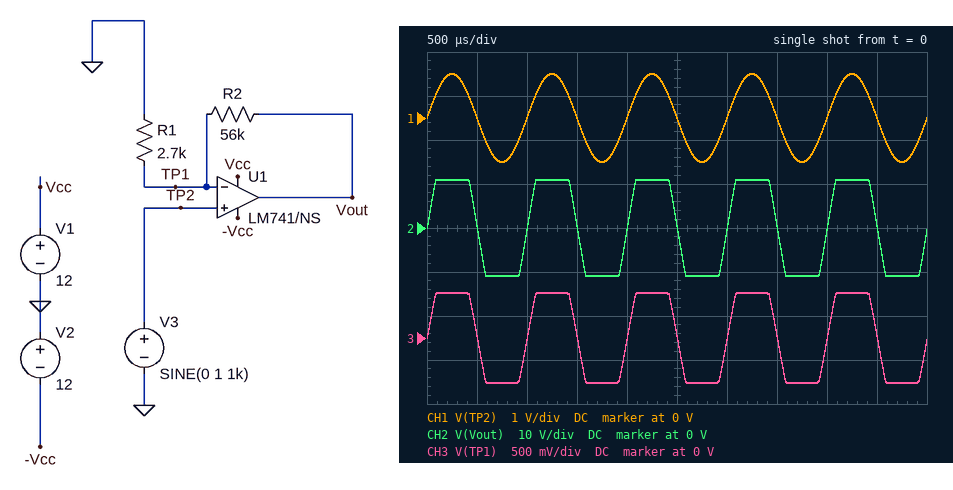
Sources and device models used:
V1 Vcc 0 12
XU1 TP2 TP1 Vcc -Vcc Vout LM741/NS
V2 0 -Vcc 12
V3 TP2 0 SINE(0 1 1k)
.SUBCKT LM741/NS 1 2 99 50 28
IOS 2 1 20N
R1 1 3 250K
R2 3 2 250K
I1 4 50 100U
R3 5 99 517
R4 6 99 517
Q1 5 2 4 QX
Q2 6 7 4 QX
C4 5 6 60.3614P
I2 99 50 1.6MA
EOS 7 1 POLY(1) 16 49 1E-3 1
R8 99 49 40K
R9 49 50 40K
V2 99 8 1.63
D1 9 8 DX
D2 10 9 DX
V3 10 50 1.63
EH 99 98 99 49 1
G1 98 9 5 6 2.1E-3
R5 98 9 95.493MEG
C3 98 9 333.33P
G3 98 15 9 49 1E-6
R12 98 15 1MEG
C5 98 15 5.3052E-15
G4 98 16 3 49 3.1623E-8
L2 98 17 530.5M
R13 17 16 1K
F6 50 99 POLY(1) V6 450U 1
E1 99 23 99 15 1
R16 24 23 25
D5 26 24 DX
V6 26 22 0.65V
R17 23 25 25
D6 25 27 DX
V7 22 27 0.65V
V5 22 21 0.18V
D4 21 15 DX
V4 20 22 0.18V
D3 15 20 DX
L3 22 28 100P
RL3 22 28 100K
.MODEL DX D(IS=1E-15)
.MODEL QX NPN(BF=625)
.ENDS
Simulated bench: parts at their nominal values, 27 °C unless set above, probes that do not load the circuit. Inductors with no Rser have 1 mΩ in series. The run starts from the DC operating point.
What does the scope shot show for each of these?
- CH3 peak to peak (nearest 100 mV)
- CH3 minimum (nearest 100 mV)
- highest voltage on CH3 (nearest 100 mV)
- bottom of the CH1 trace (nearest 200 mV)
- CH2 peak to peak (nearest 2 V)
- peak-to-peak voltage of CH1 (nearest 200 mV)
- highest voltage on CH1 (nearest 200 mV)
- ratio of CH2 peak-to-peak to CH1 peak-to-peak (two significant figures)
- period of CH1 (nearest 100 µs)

1.0 V
-500 mV
500 mV
-1.0 V
22 V
2.0 V
1.0 V
11
1.0 ms
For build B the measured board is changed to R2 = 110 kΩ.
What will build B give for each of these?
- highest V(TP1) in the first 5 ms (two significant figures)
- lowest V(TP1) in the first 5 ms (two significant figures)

270 mV
-270 mV
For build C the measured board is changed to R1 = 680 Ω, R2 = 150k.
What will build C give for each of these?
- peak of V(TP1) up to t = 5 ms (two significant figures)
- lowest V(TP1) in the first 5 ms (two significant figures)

51 mV
-51 mV
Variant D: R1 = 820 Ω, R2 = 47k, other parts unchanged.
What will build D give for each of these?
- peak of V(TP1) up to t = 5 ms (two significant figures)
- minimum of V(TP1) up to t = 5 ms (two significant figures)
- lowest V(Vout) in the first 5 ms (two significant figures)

190 mV
-190 mV
-11 V
